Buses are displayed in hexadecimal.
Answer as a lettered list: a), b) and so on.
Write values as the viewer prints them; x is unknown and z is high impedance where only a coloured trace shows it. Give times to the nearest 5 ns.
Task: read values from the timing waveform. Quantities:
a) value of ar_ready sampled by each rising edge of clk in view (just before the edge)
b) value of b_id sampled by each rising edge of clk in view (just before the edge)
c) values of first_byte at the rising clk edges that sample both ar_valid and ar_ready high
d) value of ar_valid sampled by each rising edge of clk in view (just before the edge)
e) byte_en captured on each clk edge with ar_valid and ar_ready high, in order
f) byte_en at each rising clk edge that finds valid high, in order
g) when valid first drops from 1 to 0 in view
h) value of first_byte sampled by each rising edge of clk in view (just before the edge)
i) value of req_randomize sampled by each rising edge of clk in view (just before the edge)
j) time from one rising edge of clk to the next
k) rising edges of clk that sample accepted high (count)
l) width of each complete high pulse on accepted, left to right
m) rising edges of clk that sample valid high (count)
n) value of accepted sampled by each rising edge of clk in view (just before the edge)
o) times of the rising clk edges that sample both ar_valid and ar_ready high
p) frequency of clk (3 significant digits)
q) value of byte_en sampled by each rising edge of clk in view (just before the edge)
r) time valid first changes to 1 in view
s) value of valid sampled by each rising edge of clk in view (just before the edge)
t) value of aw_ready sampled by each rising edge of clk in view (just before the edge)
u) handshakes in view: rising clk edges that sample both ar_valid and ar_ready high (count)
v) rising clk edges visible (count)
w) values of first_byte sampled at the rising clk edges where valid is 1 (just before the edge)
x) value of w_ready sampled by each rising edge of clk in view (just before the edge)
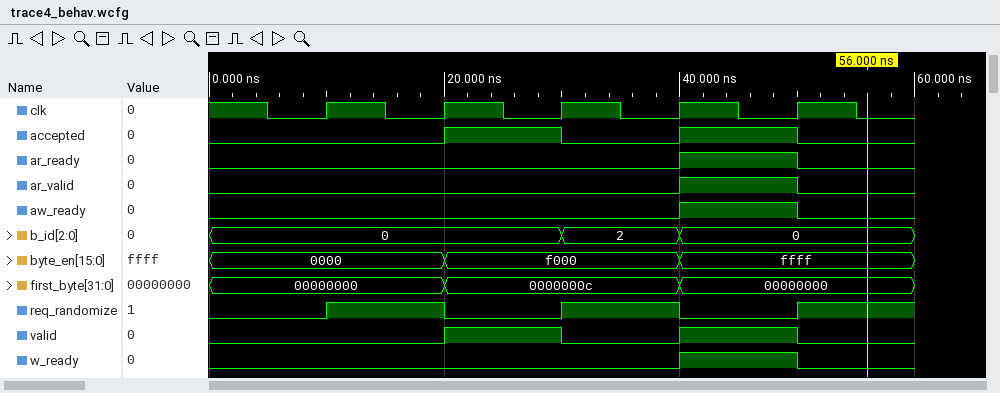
a) 0 0 0 0 1
b) 0, 0, 0, 2, 0
c) 00000000
d) 0 0 0 0 1
e) ffff
f) f000, ffff
g) 30 ns
h) 00000000, 00000000, 0000000c, 0000000c, 00000000
i) 0 1 0 1 0
j) 10 ns
k) 2
l) 10 ns, 10 ns
m) 2
n) 0 0 1 0 1
o) 50 ns
p) 100 MHz
q) 0000, 0000, f000, f000, ffff
r) 20 ns
s) 0 0 1 0 1
t) 0 0 0 0 1
u) 1
v) 5
w) 0000000c, 00000000
x) 0 0 0 0 1
